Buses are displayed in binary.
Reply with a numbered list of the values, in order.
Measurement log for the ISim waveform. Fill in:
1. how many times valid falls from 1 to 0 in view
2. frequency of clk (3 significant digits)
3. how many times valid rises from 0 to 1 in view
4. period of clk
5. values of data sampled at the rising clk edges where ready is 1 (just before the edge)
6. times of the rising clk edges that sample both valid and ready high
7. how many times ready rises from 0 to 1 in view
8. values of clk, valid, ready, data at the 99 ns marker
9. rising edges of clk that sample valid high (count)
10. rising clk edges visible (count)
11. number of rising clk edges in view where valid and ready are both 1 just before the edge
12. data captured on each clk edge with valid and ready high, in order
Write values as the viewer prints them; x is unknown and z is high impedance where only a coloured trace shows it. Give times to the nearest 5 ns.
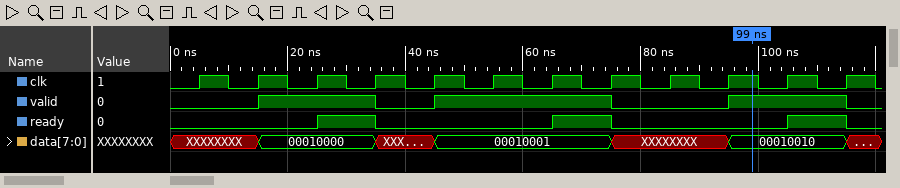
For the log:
1. 3
2. 100 MHz
3. 3
4. 10 ns
5. 00010000, 00010001, 00010010
6. 35 ns, 75 ns, 115 ns
7. 3
8. clk=1, valid=1, ready=0, data=00010010
9. 7
10. 12
11. 3
12. 00010000, 00010001, 00010010
